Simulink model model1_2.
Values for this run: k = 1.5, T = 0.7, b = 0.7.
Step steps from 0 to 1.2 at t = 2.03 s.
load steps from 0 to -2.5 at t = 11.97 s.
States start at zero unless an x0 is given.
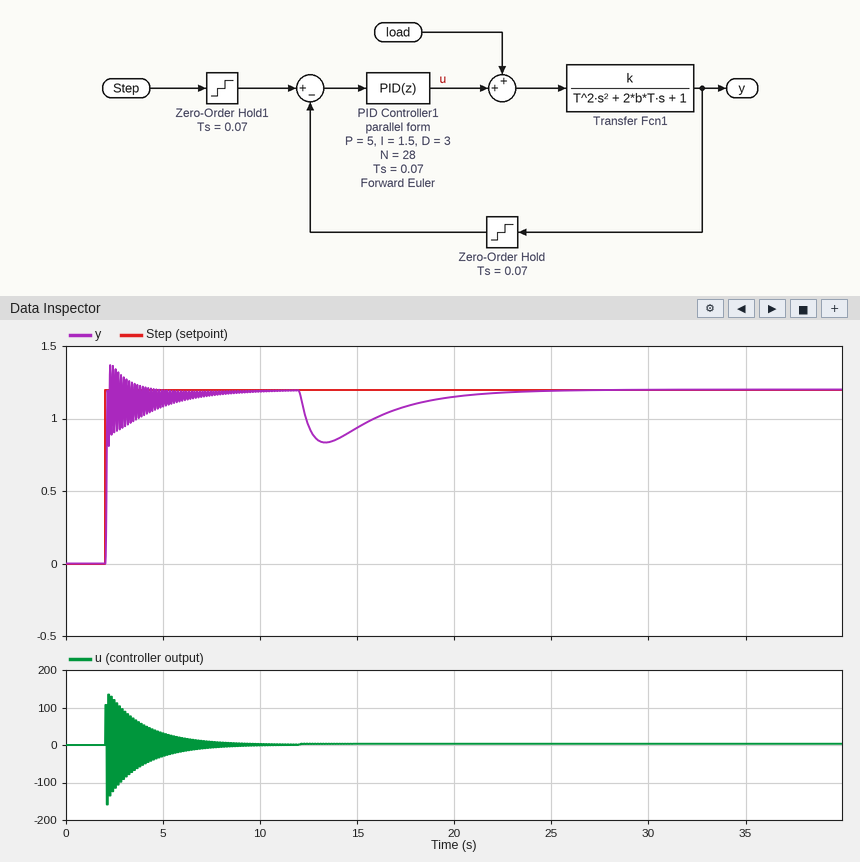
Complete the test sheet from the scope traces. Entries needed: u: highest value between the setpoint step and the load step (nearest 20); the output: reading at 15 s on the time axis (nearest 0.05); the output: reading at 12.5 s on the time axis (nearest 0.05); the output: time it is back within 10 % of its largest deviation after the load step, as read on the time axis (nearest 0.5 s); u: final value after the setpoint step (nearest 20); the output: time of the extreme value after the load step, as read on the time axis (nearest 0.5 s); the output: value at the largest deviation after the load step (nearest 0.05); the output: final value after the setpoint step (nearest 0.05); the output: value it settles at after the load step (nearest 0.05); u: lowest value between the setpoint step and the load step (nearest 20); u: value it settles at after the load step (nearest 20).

140
0.95
0.95
21.0 s
0
13.5 s
0.85
1.20
1.20
-160
0
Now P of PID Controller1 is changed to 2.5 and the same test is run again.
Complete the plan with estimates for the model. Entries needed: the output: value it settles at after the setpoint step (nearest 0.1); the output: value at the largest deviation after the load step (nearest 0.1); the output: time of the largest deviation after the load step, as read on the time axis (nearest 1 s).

1.2
0.7
14 s
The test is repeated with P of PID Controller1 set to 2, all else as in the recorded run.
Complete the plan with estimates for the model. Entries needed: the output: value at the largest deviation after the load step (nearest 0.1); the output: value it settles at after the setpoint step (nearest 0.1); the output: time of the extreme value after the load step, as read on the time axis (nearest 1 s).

0.6
1.2
14 s
